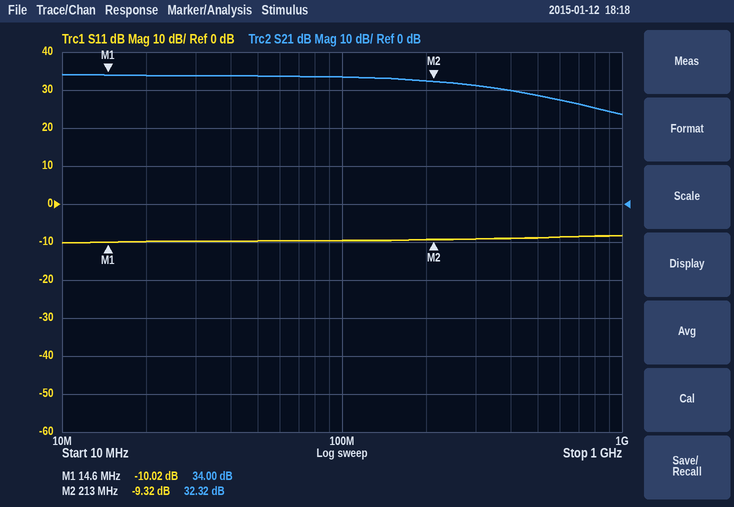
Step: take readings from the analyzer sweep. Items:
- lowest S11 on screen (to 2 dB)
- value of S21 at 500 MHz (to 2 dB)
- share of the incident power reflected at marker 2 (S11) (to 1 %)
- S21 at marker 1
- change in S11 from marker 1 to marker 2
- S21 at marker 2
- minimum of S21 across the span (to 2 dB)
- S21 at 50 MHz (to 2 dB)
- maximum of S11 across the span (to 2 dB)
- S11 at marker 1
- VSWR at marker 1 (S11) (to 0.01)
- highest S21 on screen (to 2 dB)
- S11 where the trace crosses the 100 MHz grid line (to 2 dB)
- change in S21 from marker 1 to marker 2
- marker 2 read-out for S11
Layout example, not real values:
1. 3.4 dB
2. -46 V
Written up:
1. -10 dB
2. 28 dB
3. 12 %
4. 34.00 dB
5. 0.70 dB
6. 32.32 dB
7. 24 dB
8. 34 dB
9. -8 dB
10. -10.02 dB
11. 1.92
12. 34 dB
13. -10 dB
14. -1.68 dB
15. -9.32 dB
